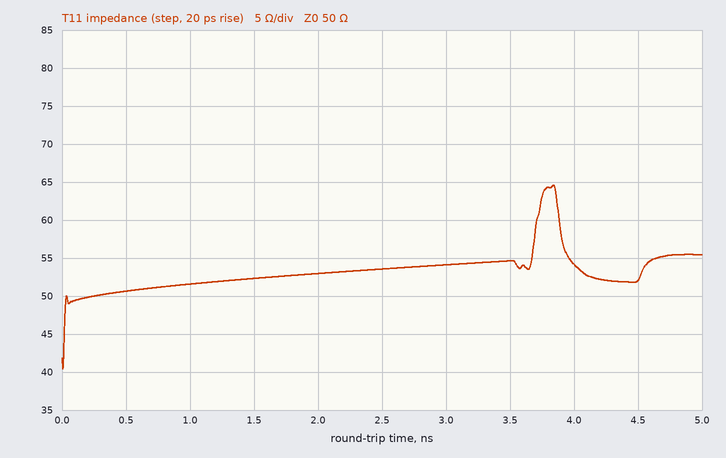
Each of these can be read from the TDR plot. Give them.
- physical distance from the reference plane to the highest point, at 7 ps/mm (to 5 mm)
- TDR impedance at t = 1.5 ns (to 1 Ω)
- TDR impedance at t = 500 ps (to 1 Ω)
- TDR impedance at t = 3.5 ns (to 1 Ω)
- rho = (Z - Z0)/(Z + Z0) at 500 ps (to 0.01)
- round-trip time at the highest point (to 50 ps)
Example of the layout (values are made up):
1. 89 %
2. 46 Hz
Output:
1. 275 mm
2. 52 Ω
3. 51 Ω
4. 55 Ω
5. +0.01
6. 3.85 ns
